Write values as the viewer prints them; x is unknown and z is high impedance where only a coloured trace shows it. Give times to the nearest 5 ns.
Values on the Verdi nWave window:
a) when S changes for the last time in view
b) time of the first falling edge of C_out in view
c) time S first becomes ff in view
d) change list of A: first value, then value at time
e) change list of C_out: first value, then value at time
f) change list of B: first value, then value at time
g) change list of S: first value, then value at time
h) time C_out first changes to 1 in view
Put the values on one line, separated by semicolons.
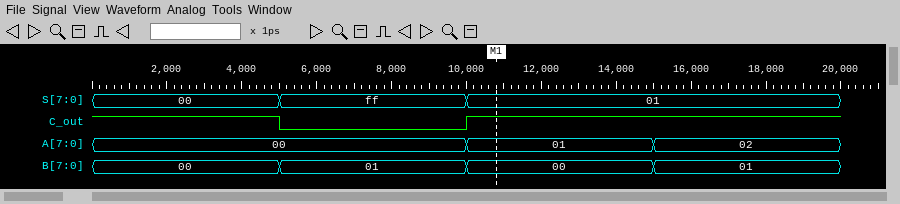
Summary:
10 ns; 5 ns; 5 ns; 00, 01 at 10 ns, 02 at 15 ns; 1, 0 at 5 ns, 1 at 10 ns; 00, 01 at 5 ns, 00 at 10 ns, 01 at 15 ns; 00, ff at 5 ns, 01 at 10 ns; 10 ns
